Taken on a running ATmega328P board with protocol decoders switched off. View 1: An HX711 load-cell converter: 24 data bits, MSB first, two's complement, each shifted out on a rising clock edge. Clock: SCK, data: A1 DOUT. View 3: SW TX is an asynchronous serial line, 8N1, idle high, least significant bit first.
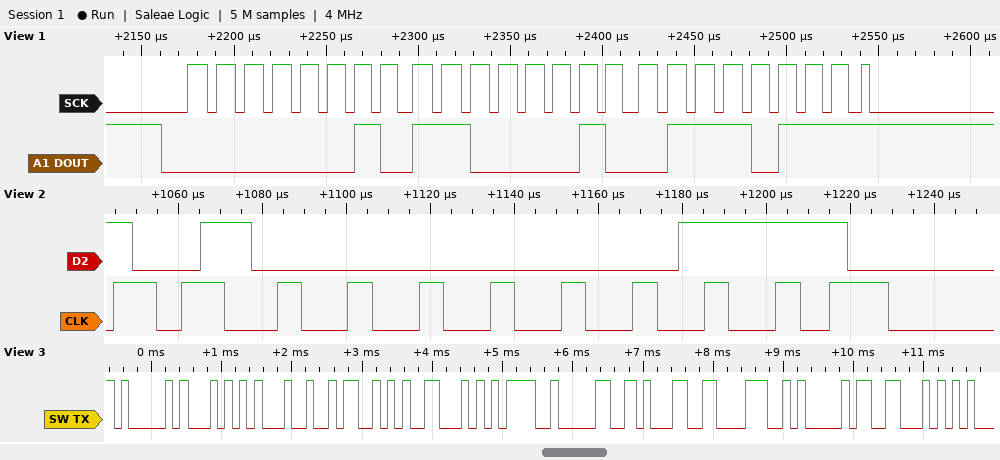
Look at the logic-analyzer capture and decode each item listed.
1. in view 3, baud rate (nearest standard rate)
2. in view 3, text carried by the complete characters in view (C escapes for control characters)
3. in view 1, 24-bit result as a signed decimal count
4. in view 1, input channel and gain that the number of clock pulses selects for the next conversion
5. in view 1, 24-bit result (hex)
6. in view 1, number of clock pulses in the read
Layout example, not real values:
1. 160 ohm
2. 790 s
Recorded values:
1. 9600 baud
2. "AT$SF=018AF"
3. 180855
4. channel A, gain 128
5. 0x02C277
6. 25
